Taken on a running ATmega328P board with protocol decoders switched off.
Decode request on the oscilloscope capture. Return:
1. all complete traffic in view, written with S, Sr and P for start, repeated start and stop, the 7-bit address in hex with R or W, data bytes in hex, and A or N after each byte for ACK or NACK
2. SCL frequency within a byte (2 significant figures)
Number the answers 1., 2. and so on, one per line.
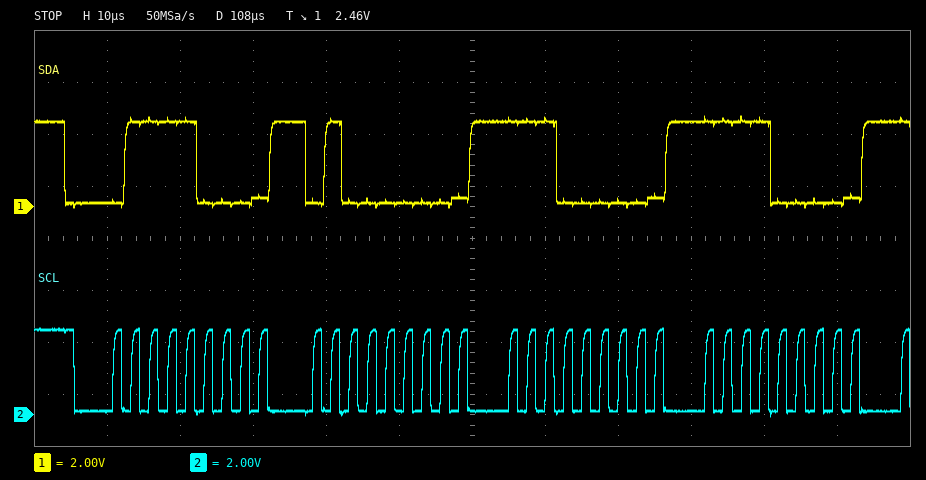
1. S 3CW A 40 A E0 A F0 A
2. 400 kHz
